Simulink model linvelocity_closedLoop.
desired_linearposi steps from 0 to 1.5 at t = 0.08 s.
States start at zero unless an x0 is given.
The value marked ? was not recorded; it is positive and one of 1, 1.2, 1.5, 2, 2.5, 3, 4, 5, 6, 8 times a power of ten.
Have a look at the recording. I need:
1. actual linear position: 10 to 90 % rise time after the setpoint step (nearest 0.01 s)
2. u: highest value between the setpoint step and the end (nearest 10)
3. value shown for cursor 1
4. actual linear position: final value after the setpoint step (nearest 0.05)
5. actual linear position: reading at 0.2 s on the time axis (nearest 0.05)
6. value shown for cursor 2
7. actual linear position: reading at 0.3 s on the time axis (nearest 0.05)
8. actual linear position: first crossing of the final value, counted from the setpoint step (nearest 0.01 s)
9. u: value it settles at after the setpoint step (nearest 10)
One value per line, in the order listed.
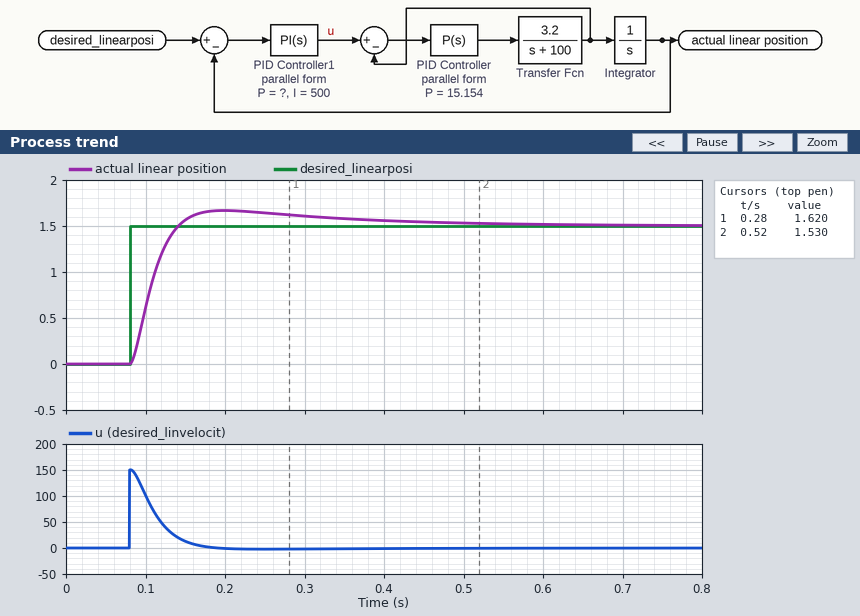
0.04 s
150
1.620
1.50
1.65
1.530
1.60
0.06 s
0
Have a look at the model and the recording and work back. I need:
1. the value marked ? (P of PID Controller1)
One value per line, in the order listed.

100
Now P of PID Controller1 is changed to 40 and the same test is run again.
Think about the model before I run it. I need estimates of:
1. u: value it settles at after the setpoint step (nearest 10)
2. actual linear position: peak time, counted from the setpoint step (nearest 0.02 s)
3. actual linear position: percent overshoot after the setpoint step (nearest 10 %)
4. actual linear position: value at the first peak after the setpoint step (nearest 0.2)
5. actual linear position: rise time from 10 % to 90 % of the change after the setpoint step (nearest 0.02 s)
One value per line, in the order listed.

0
0.18 s
30 %
2.0
0.06 s
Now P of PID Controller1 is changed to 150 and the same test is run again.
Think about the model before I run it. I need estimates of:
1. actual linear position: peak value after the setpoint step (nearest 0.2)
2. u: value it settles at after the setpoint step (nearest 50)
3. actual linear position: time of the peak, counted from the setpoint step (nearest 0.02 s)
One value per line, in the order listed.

1.6
0
0.08 s
